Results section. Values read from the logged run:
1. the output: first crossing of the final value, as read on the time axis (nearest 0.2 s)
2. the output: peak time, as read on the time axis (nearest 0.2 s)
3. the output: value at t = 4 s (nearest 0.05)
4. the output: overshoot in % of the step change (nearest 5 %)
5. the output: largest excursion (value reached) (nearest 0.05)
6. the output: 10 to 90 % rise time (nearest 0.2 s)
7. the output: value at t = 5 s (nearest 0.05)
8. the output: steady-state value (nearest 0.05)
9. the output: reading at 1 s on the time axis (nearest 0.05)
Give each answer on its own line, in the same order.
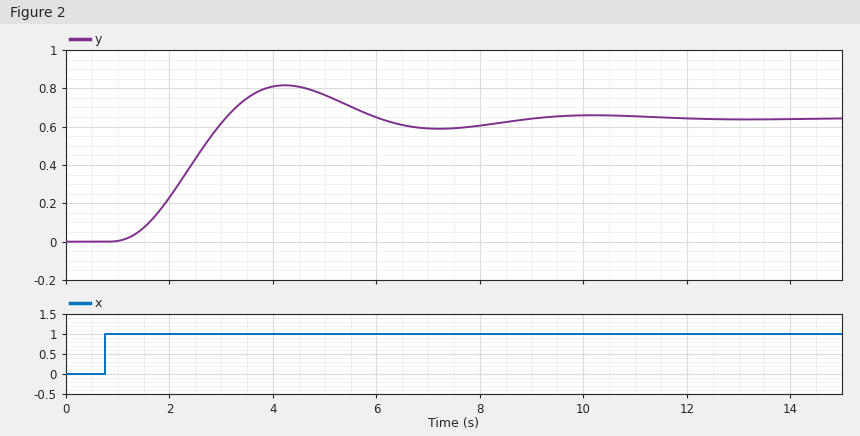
3.0 s
4.2 s
0.80
25 %
0.80
1.4 s
0.75
0.65
0.00
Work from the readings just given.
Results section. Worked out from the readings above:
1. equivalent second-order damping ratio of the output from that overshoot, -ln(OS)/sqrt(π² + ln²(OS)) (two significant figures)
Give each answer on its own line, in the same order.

0.40
